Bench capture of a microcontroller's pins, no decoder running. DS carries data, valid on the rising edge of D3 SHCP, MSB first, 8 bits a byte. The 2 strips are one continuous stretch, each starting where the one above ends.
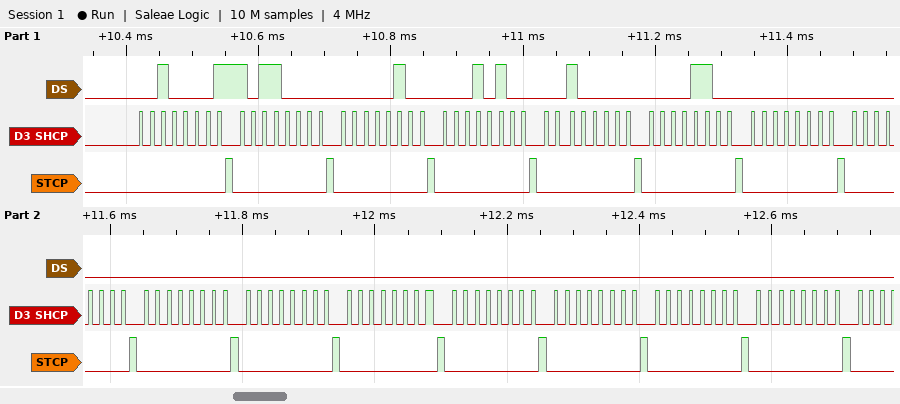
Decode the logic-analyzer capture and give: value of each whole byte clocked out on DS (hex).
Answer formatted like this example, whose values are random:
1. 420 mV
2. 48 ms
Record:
1. 21 B0 04 14 20 0C 00 00 00 00 00 00 00 00 00
